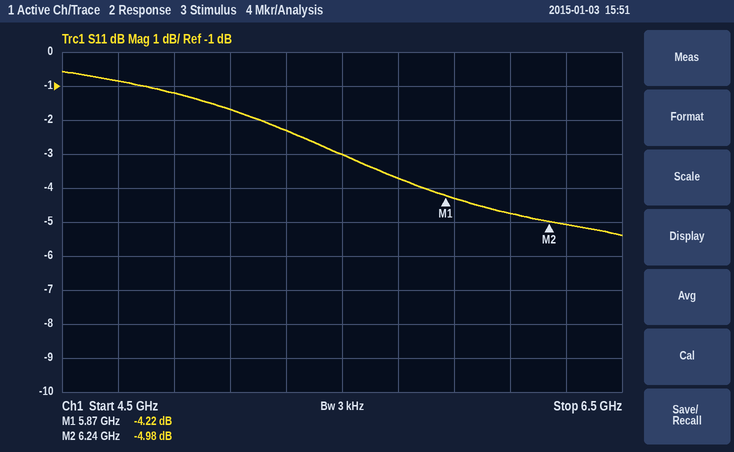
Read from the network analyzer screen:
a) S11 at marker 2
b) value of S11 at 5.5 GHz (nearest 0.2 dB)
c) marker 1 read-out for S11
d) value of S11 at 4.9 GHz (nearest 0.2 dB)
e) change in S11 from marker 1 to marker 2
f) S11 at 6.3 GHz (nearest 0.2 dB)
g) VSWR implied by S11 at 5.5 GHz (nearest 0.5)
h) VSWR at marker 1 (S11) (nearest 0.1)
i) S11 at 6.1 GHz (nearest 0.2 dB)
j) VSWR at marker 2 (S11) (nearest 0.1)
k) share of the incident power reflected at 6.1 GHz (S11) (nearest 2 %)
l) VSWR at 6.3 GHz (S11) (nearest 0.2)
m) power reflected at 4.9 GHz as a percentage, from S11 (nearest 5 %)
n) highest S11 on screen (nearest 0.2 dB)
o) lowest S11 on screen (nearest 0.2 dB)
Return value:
-4.98 dB
-3.0 dB
-4.22 dB
-1.2 dB
-0.76 dB
-5.0 dB
6.0
4.2
-4.8 dB
3.6
34 %
3.6
75 %
-0.6 dB
-5.4 dB
